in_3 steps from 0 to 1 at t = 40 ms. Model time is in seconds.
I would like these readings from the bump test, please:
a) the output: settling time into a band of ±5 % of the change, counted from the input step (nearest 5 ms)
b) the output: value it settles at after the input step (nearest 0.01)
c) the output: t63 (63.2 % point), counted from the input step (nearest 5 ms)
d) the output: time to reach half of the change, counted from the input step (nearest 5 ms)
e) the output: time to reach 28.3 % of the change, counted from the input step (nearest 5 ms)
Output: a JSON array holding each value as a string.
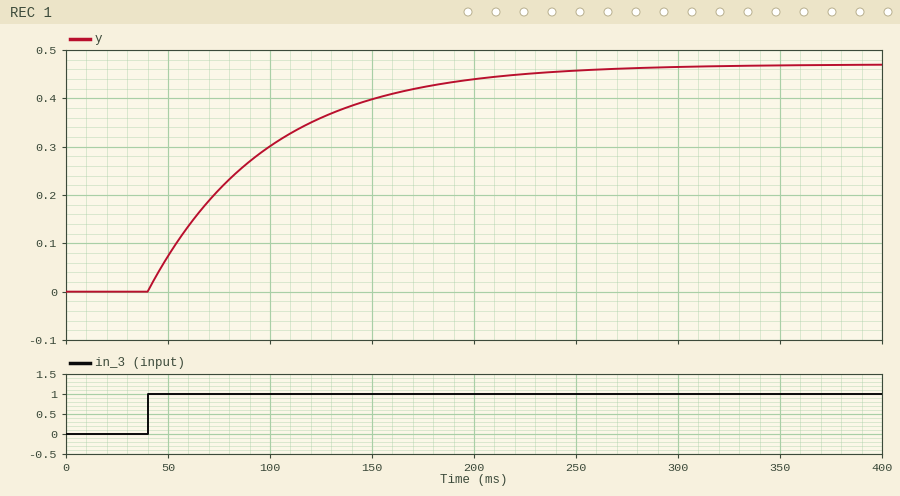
["175 ms", "0.47", "60 ms", "40 ms", "20 ms"]
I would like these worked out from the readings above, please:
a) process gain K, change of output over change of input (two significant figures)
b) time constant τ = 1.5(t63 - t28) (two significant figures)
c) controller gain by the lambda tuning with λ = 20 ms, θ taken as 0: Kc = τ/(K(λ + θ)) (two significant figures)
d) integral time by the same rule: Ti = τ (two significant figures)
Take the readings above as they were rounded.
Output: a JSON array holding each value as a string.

["0.47", "60 ms", "6.4", "60 ms"]
